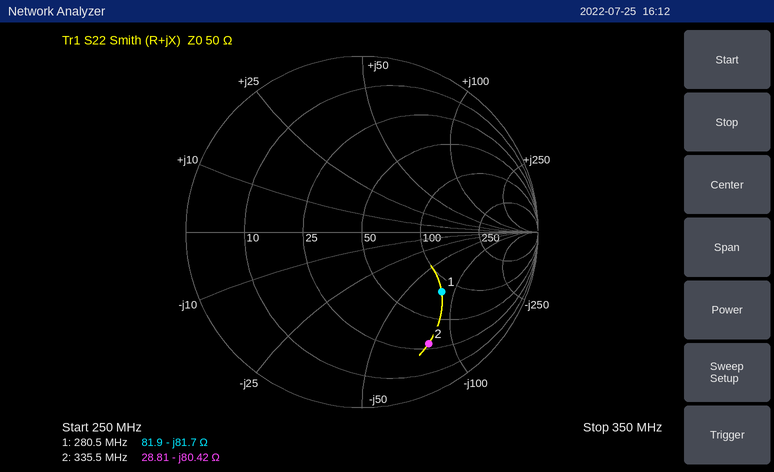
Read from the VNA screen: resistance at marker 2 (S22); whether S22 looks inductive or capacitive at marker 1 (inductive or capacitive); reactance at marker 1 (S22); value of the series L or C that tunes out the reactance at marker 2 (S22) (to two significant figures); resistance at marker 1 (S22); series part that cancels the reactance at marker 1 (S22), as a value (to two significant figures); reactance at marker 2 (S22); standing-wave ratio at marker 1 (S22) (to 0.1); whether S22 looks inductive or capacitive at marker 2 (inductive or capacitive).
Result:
28.81 Ω
capacitive
-81.7 Ω
38 nH
81.9 Ω
46 nH
-80.42 Ω
3.6
capacitive
